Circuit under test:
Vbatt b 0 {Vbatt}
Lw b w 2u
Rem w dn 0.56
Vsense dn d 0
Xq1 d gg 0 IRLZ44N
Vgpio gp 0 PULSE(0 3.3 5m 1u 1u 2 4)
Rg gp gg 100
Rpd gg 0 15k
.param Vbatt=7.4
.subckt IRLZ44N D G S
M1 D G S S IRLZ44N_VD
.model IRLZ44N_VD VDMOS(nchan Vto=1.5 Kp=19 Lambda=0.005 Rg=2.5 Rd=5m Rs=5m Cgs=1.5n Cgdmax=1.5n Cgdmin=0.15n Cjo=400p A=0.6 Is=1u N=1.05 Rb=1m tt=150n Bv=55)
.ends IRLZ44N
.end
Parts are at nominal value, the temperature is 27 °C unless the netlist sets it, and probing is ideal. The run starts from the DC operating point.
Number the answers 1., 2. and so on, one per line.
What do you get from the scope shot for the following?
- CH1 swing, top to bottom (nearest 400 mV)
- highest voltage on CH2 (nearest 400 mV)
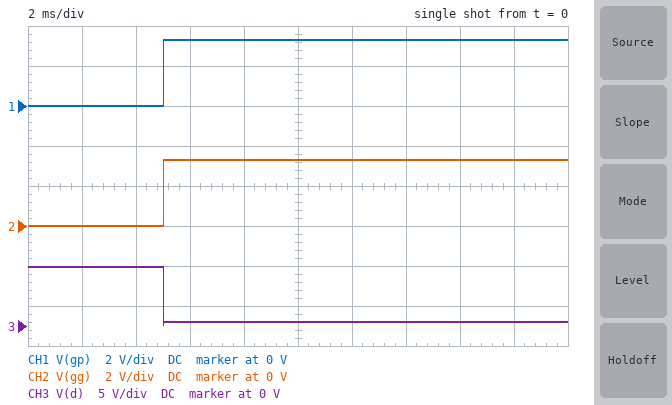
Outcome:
1. 3.2 V
2. 3.2 V
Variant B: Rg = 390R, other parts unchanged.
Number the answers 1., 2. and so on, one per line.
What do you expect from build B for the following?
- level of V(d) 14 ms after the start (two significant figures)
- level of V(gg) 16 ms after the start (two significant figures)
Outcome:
1. 570 mV
2. 3.2 V
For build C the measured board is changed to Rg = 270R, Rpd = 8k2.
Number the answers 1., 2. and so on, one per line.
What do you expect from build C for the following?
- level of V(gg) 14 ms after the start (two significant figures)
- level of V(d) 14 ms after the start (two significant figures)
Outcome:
1. 3.2 V
2. 580 mV
